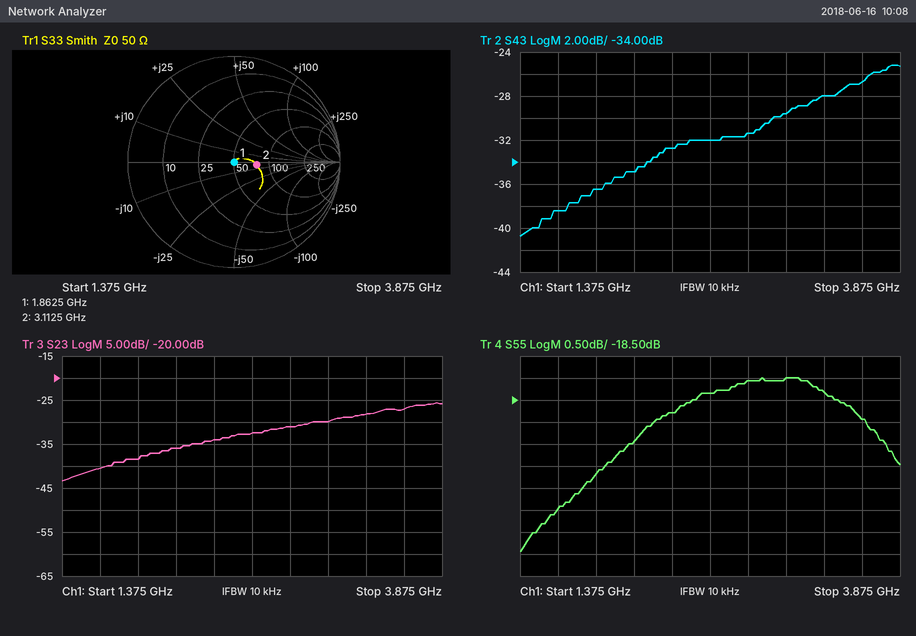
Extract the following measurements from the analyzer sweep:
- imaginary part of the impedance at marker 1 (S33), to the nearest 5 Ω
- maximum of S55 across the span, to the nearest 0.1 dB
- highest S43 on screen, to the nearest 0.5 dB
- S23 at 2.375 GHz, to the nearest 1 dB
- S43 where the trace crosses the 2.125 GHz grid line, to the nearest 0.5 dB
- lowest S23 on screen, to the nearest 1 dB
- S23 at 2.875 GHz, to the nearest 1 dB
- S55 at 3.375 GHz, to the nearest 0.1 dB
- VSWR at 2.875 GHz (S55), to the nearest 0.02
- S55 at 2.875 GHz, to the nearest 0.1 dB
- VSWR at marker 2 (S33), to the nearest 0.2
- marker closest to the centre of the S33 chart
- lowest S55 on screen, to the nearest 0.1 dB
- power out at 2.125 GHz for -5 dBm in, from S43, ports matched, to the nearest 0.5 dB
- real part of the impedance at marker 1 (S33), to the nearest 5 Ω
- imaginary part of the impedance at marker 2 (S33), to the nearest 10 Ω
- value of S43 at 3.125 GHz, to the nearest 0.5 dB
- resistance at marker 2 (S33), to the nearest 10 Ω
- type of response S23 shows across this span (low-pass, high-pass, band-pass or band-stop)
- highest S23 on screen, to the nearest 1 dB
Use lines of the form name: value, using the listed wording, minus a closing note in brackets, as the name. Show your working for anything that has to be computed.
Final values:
imaginary part of the impedance at marker 1 (S33), to the nearest 5 Ω: 0 Ω
maximum of S55 across the span, to the nearest 0.1 dB: -18.0 dB
highest S43 on screen, to the nearest 0.5 dB: -25.0 dB
S23 at 2.375 GHz, to the nearest 1 dB: -34 dB
S43 where the trace crosses the 2.125 GHz grid line, to the nearest 0.5 dB: -35.0 dB
lowest S23 on screen, to the nearest 1 dB: -43 dB
S23 at 2.875 GHz, to the nearest 1 dB: -31 dB
S55 at 3.375 GHz, to the nearest 0.1 dB: -18.3 dB
VSWR at 2.875 GHz (S55), to the nearest 0.02: |Γ| = 10^(-18.1/20) = 0.1245; VSWR = (1 + 0.1245)/(1 − 0.1245) ≈ 1.28
S55 at 2.875 GHz, to the nearest 0.1 dB: -18.1 dB
VSWR at marker 2 (S33), to the nearest 0.2: 1.6
marker closest to the centre of the S33 chart: marker 1
lowest S55 on screen, to the nearest 0.1 dB: -21.9 dB
power out at 2.125 GHz for -5 dBm in, from S43, ports matched, to the nearest 0.5 dB: -5 dBm + (-35.0 dB) = -40.0 dBm
real part of the impedance at marker 1 (S33), to the nearest 5 Ω: 50 Ω
imaginary part of the impedance at marker 2 (S33), to the nearest 10 Ω: 0 Ω
value of S43 at 3.125 GHz, to the nearest 0.5 dB: -29.5 dB
resistance at marker 2 (S33), to the nearest 10 Ω: 80 Ω
type of response S23 shows across this span: high-pass
highest S23 on screen, to the nearest 1 dB: -26 dB
